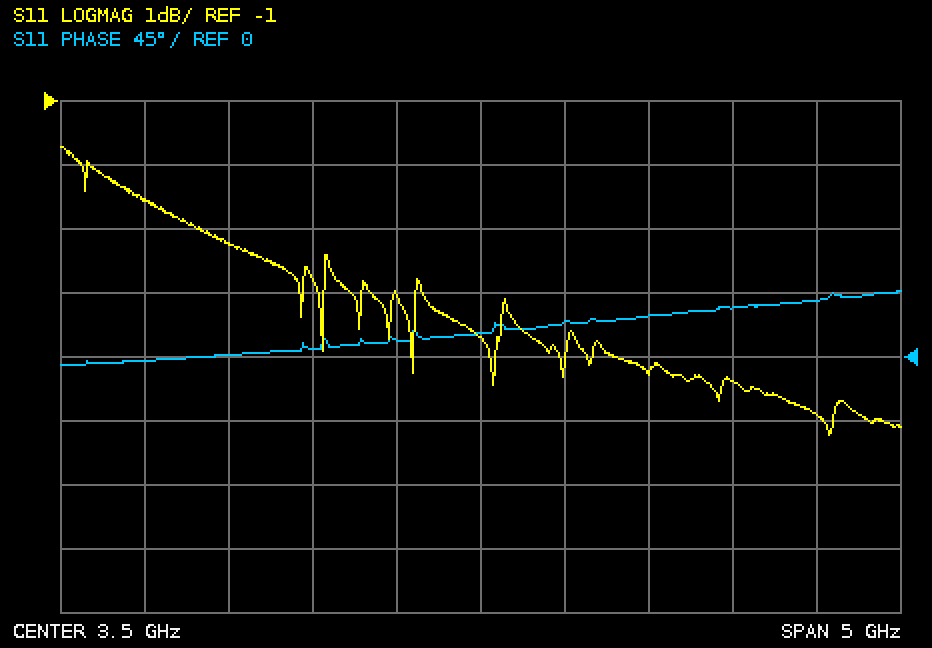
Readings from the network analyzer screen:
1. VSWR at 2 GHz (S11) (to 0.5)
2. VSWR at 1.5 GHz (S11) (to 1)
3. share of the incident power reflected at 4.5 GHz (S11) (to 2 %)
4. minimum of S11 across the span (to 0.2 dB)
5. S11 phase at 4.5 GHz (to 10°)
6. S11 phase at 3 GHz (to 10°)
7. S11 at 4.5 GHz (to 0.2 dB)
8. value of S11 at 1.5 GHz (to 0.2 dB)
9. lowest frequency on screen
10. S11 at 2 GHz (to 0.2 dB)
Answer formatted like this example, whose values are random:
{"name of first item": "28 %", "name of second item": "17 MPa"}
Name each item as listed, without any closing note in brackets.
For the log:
{"VSWR at 2 GHz (S11)": "5.5", "VSWR at 1.5 GHz (S11)": "7", "share of the incident power reflected at 4.5 GHz (S11)": "30 %", "minimum of S11 across the span": "-6.2 dB", "S11 phase at 4.5 GHz": "30°", "S11 phase at 3 GHz": "10°", "S11 at 4.5 GHz": "-5.2 dB", "value of S11 at 1.5 GHz": "-2.6 dB", "lowest frequency on screen": "1 GHz", "S11 at 2 GHz": "-3.2 dB"}
